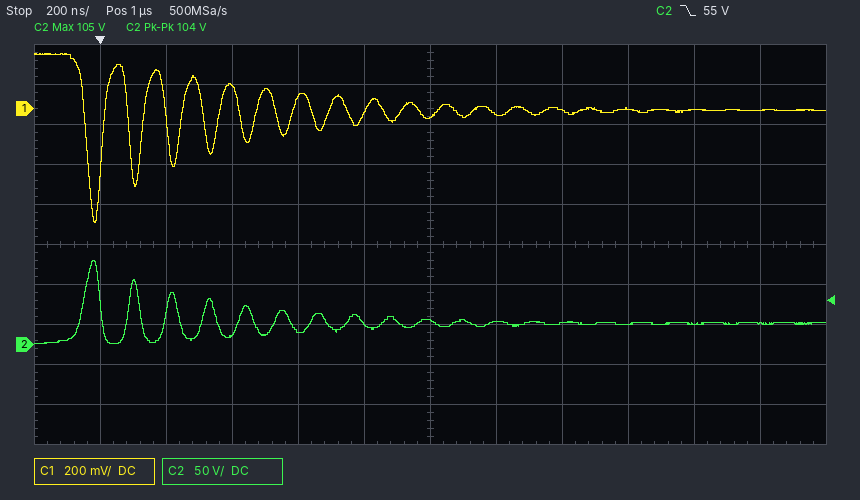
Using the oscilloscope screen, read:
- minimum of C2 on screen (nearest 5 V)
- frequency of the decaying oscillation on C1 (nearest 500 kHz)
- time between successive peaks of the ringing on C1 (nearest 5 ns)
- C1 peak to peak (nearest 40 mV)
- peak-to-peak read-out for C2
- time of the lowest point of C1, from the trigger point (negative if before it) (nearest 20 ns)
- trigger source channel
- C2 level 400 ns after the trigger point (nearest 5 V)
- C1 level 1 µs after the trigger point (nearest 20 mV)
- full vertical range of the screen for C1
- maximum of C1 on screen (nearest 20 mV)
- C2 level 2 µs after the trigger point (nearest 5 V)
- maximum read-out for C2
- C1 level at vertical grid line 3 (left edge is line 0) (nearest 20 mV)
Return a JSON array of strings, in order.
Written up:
["0 V", "9.0 MHz", "110 ns", "840 mV", "104 V", "-20 ns", "C2", "15 V", "-40 mV", "2 V", "280 mV", "25 V", "105 V", "100 mV"]
